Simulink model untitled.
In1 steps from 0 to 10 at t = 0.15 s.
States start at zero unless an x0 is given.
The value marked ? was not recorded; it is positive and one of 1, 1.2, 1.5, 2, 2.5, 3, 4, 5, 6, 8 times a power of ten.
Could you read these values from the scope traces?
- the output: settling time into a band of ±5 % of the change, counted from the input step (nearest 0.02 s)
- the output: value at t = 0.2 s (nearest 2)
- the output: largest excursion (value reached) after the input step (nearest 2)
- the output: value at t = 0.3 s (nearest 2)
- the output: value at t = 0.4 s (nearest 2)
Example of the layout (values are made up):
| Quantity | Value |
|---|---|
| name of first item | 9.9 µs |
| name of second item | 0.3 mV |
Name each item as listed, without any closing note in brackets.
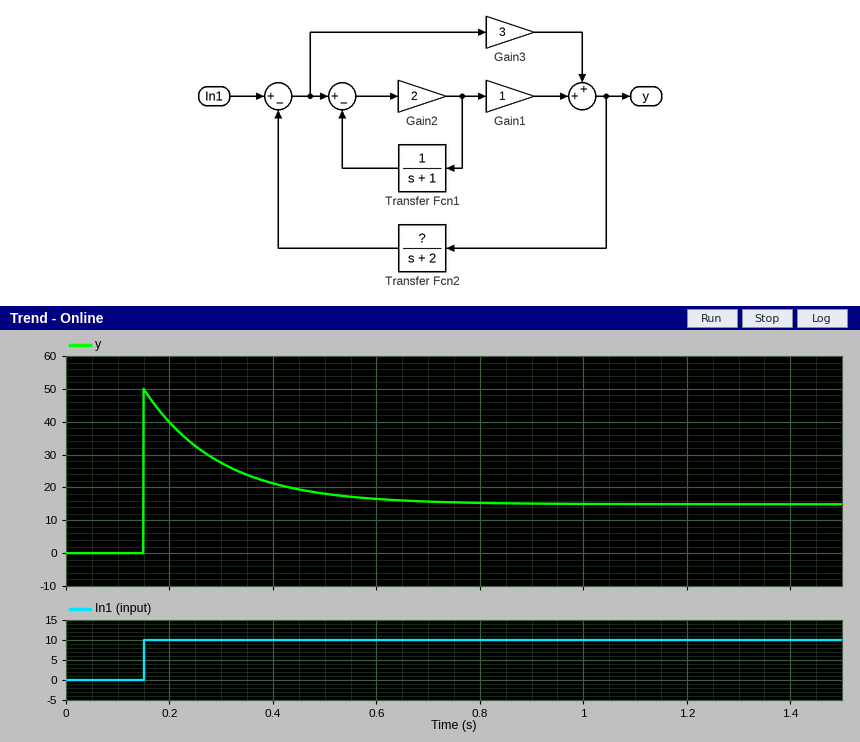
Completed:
| Quantity | Value |
|---|---|
| the output: settling time into a band of ±5 % of the change, counted from the input step | 0.56 s |
| the output: value at t = 0.2 s | 40 |
| the output: largest excursion (value reached) after the input step | 50 |
| the output: value at t = 0.3 s | 28 |
| the output: value at t = 0.4 s | 22 |
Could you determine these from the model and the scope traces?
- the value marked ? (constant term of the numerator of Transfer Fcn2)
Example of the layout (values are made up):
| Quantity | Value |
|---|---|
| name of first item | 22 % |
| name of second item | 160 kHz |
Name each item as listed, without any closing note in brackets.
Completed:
| Quantity | Value |
|---|---|
| the value marked ? | 0.8 |
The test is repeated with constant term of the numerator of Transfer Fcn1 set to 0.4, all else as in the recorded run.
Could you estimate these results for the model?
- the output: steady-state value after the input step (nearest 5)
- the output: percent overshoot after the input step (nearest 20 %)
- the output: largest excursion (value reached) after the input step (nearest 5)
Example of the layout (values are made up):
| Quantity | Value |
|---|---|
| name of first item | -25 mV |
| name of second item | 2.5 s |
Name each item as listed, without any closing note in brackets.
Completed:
| Quantity | Value |
|---|---|
| the output: steady-state value after the input step | 15 |
| the output: percent overshoot after the input step | 220 % |
| the output: largest excursion (value reached) after the input step | 50 |
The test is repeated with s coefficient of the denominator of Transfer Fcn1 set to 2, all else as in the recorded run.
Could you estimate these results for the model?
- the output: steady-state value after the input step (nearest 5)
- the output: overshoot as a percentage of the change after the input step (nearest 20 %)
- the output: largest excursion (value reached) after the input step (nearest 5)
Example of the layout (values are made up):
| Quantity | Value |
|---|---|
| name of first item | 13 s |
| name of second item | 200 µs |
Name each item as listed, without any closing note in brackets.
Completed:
| Quantity | Value |
|---|---|
| the output: steady-state value after the input step | 15 |
| the output: overshoot as a percentage of the change after the input step | 240 % |
| the output: largest excursion (value reached) after the input step | 50 |
